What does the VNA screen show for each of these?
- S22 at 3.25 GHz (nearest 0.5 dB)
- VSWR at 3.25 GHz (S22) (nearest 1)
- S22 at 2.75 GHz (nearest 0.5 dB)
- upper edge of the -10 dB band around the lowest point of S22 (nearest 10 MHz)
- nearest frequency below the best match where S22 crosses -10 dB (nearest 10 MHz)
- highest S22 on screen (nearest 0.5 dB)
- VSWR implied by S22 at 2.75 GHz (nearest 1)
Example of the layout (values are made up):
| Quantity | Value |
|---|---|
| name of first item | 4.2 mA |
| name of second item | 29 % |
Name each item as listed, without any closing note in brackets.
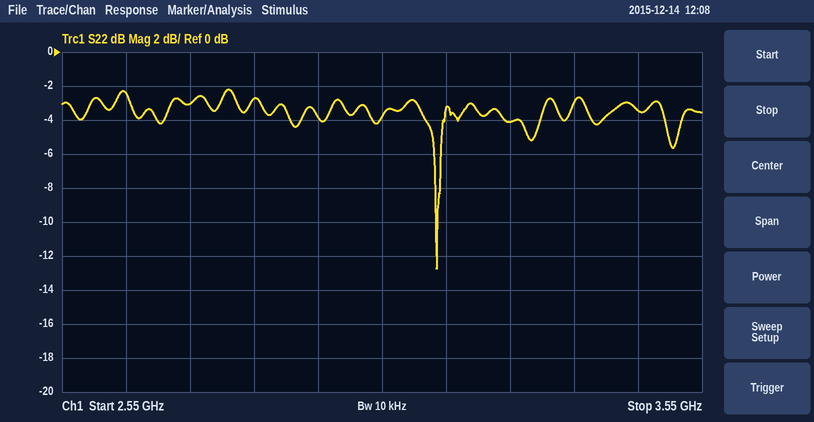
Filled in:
| Quantity | Value |
|---|---|
| S22 at 3.25 GHz | -4.0 dB |
| VSWR at 3.25 GHz (S22) | 4 |
| S22 at 2.75 GHz | -3.0 dB |
| upper edge of the -10 dB band around the lowest point of S22 | 3.14 GHz |
| nearest frequency below the best match where S22 crosses -10 dB | 3.13 GHz |
| highest S22 on screen | -2.0 dB |
| VSWR implied by S22 at 2.75 GHz | 6 |
